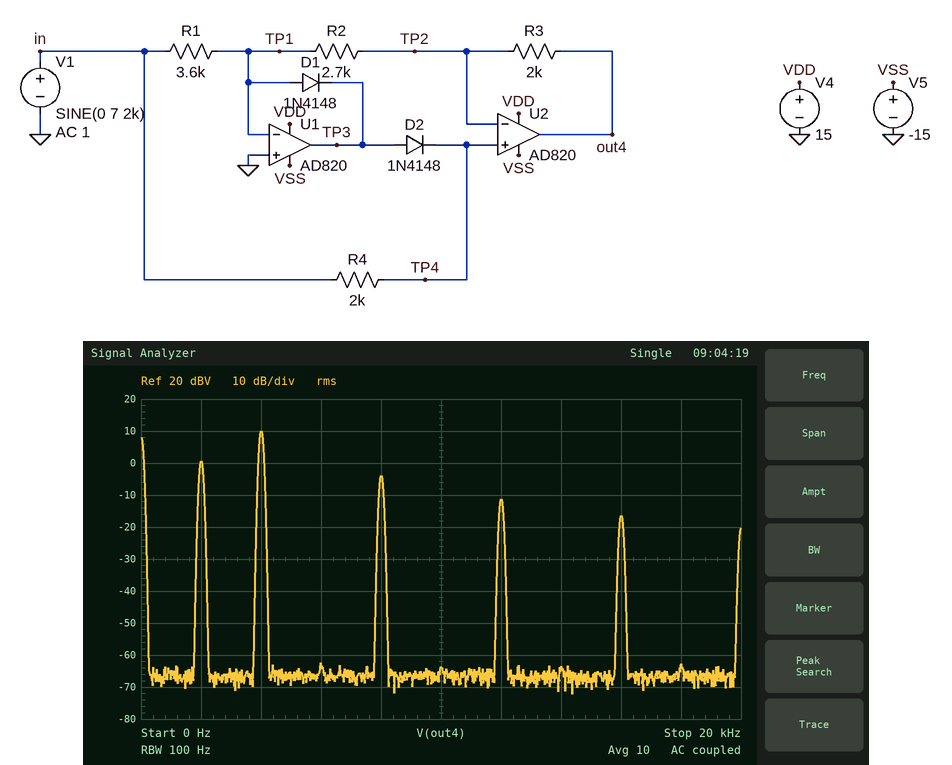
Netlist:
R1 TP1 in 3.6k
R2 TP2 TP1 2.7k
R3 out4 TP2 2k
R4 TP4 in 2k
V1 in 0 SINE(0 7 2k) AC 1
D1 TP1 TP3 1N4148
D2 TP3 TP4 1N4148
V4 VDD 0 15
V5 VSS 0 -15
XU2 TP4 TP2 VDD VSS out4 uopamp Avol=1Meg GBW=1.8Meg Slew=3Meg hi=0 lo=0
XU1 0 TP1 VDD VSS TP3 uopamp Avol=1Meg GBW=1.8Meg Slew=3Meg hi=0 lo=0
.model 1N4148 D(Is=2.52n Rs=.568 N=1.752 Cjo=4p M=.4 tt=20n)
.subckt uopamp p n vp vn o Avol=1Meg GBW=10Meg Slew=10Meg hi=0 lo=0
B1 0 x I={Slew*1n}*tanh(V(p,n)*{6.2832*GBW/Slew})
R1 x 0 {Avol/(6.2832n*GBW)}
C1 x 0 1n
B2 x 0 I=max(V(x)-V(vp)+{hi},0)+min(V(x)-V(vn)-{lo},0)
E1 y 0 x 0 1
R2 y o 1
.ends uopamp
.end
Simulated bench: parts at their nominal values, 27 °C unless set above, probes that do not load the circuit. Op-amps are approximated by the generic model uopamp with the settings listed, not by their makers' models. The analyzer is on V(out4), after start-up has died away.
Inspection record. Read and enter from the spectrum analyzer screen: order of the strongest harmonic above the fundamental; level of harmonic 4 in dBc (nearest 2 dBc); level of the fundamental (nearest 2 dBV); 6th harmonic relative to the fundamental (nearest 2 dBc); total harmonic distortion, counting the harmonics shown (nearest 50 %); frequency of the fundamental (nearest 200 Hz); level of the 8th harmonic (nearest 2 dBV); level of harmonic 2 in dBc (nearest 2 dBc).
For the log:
2
-4 dBc
0 dBV
-12 dBc
300 %
2.0 kHz
-16 dBV
10 dBc
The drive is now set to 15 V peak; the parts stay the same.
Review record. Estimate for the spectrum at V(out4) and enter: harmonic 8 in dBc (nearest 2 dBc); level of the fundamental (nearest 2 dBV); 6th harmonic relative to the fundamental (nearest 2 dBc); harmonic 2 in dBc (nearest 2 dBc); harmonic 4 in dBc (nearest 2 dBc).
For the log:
-4 dBc
-10 dBV
8 dBc
22 dBc
16 dBc
